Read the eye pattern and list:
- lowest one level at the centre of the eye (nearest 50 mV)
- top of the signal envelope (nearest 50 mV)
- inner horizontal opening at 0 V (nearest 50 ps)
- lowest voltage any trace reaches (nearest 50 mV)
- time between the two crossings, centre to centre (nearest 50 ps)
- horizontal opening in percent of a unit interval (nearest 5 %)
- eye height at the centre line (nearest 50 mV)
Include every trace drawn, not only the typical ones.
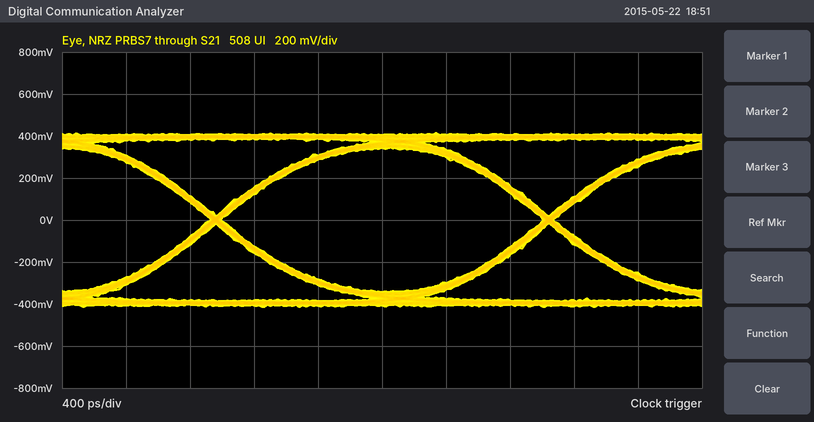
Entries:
350 mV
400 mV
2.00 ns
-400 mV
2.10 ns
95 %
700 mV
